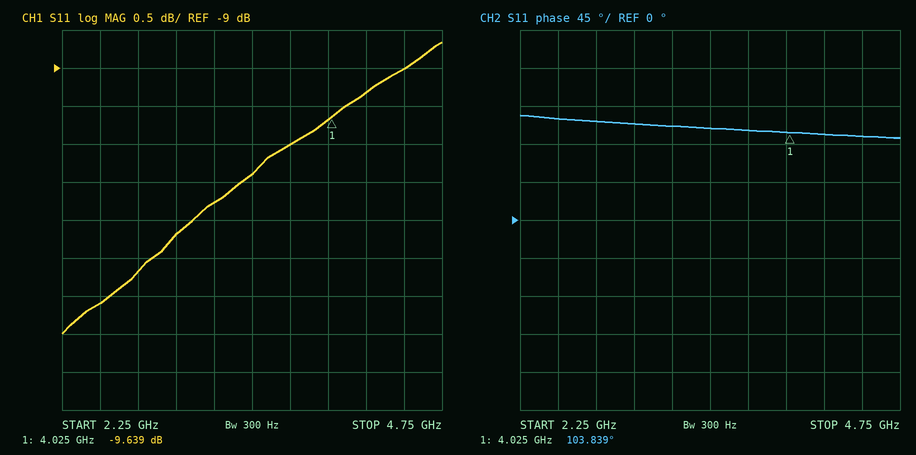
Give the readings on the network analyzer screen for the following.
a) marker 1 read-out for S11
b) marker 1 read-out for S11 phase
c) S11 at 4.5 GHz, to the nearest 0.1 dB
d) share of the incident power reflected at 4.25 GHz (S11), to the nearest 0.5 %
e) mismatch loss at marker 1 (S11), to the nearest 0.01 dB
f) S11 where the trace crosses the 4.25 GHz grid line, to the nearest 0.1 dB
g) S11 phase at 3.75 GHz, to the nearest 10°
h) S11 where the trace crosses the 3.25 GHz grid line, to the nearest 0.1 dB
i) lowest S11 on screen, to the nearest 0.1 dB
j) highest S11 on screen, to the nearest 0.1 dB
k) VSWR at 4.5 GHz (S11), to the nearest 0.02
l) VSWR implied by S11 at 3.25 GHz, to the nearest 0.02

-9.639 dB
103.839°
-9.0 dB
11.5 %
0.50 dB
-9.3 dB
110°
-10.8 dB
-12.5 dB
-8.7 dB
2.10
1.82
